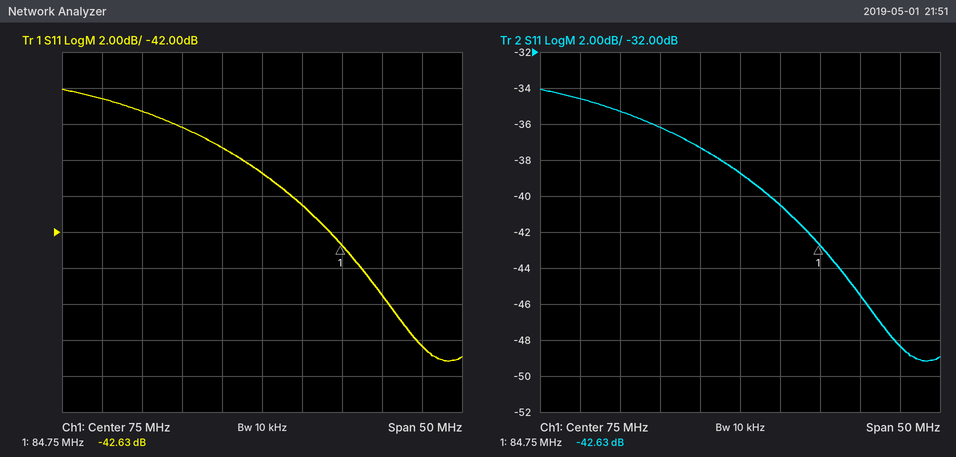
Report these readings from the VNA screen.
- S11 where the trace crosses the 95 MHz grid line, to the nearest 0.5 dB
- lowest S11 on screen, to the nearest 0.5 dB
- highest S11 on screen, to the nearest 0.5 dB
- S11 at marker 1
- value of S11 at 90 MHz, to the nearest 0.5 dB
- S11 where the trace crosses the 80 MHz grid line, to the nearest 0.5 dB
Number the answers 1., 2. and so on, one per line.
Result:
1. -48.5 dB
2. -49.0 dB
3. -34.0 dB
4. -42.63 dB
5. -45.5 dB
6. -40.5 dB
